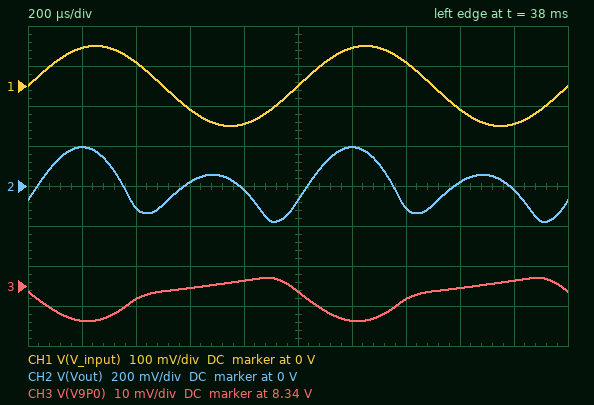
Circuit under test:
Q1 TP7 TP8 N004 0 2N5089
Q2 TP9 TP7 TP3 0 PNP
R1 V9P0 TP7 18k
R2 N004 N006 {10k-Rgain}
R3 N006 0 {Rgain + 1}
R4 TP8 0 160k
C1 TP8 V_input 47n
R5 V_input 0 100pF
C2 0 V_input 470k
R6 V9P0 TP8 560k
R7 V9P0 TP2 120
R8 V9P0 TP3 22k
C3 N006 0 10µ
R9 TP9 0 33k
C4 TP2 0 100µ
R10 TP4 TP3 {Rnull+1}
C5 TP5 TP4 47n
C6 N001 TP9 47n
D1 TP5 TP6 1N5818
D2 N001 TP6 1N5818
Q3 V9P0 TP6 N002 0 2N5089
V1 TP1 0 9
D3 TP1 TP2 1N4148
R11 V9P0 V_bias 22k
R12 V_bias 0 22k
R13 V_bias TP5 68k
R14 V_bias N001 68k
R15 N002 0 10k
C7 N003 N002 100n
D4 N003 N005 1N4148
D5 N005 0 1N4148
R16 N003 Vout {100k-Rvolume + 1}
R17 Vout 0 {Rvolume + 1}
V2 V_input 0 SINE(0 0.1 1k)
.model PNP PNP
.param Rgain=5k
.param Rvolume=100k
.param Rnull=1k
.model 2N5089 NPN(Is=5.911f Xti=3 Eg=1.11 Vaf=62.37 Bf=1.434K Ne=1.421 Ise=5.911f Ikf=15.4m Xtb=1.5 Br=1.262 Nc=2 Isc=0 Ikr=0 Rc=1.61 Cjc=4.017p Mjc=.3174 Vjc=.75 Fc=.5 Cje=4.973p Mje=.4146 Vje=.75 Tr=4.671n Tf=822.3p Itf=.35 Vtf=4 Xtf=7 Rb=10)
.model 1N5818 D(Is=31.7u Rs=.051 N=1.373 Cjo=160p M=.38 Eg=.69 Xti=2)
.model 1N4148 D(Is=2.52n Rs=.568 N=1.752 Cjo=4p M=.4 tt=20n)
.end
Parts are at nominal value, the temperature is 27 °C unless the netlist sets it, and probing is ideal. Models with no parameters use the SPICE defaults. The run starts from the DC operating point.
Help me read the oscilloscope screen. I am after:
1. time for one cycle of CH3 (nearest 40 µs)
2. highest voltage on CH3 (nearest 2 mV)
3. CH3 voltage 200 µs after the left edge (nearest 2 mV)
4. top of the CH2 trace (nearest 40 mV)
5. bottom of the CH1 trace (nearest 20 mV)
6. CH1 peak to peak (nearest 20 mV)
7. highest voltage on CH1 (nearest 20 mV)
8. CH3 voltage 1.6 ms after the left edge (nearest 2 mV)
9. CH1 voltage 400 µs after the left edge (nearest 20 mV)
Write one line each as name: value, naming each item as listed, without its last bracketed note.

time for one cycle of CH3: 1.00 ms
highest voltage on CH3: 8.342 V
CH3 voltage 200 µs after the left edge: 8.332 V
top of the CH2 trace: 200 mV
bottom of the CH1 trace: -100 mV
CH1 peak to peak: 200 mV
highest voltage on CH1: 100 mV
CH3 voltage 1.6 ms after the left edge: 8.340 V
CH1 voltage 400 µs after the left edge: 60 mV
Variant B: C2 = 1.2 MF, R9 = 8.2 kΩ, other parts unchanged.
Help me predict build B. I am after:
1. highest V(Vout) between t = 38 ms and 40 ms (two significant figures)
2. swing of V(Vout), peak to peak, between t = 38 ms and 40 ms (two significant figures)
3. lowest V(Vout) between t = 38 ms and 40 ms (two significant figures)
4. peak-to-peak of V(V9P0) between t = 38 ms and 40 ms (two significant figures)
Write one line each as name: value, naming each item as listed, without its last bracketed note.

highest V(Vout) between t = 38 ms and 40 ms: 120 mV
swing of V(Vout), peak to peak, between t = 38 ms and 40 ms: 250 mV
lowest V(Vout) between t = 38 ms and 40 ms: -130 mV
peak-to-peak of V(V9P0) between t = 38 ms and 40 ms: 6.9 mV
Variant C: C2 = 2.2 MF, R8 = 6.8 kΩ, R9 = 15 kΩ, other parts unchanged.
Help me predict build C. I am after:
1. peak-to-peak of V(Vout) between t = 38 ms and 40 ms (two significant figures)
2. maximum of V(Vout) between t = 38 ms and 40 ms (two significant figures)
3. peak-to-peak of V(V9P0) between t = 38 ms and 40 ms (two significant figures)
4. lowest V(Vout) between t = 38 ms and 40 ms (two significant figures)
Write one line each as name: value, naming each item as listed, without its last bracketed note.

peak-to-peak of V(Vout) between t = 38 ms and 40 ms: 630 mV
maximum of V(Vout) between t = 38 ms and 40 ms: 340 mV
peak-to-peak of V(V9P0) between t = 38 ms and 40 ms: 20 mV
lowest V(Vout) between t = 38 ms and 40 ms: -290 mV
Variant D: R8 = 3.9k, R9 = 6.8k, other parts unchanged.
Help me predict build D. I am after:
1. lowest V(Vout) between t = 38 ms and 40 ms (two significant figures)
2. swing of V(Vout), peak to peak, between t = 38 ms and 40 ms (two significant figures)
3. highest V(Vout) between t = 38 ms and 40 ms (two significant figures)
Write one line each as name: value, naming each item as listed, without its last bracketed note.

lowest V(Vout) between t = 38 ms and 40 ms: -240 mV
swing of V(Vout), peak to peak, between t = 38 ms and 40 ms: 500 mV
highest V(Vout) between t = 38 ms and 40 ms: 260 mV
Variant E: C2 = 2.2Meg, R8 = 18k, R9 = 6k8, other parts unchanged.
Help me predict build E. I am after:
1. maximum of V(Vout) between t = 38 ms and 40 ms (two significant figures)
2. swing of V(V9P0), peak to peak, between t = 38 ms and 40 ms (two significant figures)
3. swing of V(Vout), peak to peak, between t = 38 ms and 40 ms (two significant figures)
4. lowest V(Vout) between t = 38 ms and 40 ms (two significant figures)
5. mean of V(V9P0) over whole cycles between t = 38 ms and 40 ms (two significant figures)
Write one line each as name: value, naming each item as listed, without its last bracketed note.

maximum of V(Vout) between t = 38 ms and 40 ms: 130 mV
swing of V(V9P0), peak to peak, between t = 38 ms and 40 ms: 7.6 mV
swing of V(Vout), peak to peak, between t = 38 ms and 40 ms: 260 mV
lowest V(Vout) between t = 38 ms and 40 ms: -130 mV
mean of V(V9P0) over whole cycles between t = 38 ms and 40 ms: 8.3 V
